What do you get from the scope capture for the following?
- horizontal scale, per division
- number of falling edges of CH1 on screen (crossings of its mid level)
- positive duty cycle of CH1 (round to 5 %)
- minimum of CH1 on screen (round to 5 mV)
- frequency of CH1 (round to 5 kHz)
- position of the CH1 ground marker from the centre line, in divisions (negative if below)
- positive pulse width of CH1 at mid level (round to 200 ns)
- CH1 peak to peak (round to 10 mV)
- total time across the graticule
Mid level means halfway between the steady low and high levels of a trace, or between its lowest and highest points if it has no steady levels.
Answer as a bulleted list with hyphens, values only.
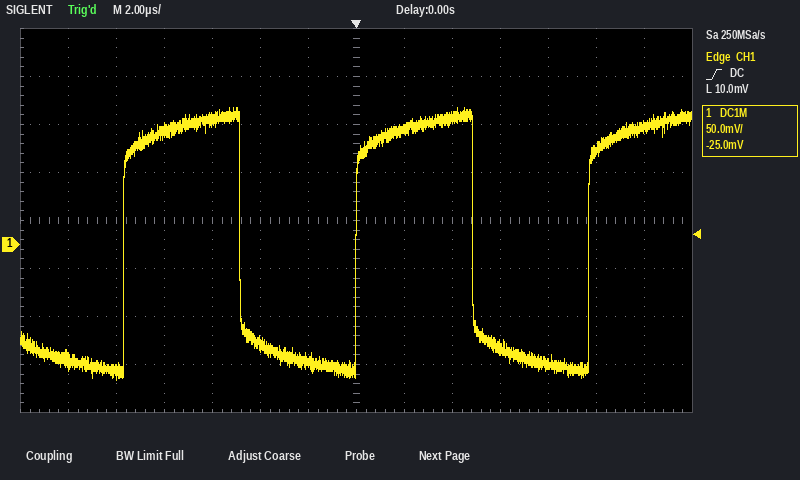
- 2 µs
- 2
- 50 %
- -140 mV
- 105 kHz
- -0.5 div
- 4.8 µs
- 280 mV
- 28 µs
